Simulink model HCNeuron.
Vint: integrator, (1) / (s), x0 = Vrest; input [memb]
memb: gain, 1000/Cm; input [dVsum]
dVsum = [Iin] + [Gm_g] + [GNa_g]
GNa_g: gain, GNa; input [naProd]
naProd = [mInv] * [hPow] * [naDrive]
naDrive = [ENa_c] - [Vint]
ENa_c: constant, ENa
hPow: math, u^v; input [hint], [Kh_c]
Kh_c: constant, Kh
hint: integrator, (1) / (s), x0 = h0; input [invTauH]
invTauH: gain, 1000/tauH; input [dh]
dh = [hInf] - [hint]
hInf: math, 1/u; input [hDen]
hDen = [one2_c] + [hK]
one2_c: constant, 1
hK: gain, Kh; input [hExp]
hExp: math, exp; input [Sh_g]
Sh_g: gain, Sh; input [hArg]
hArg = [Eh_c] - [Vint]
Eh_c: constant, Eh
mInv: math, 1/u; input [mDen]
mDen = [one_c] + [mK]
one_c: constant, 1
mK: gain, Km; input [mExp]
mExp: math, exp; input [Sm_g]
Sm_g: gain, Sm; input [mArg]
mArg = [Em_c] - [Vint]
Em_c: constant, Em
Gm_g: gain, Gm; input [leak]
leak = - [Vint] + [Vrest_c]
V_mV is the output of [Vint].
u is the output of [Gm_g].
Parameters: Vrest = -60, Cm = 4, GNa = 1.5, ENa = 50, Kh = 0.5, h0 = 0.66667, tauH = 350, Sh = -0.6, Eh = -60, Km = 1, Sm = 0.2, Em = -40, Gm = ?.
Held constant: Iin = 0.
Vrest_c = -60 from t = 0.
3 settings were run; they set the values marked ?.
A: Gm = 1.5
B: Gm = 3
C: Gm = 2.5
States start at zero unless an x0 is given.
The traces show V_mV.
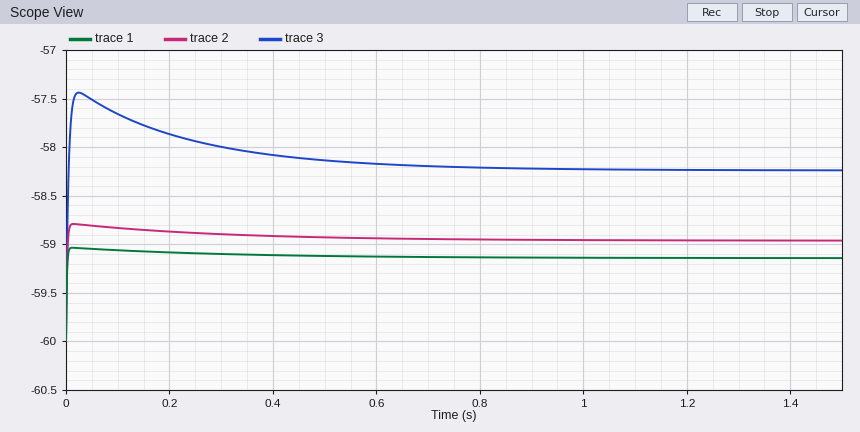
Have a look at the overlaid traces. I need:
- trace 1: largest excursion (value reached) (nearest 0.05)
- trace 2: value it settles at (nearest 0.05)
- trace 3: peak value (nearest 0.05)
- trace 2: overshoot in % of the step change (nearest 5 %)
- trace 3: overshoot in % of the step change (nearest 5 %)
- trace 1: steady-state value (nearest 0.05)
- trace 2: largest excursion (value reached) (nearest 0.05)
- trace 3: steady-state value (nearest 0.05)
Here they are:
-59.05
-58.95
-57.45
15 %
45 %
-59.15
-58.80
-58.25
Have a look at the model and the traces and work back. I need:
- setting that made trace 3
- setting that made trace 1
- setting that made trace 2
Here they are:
A
B
C
